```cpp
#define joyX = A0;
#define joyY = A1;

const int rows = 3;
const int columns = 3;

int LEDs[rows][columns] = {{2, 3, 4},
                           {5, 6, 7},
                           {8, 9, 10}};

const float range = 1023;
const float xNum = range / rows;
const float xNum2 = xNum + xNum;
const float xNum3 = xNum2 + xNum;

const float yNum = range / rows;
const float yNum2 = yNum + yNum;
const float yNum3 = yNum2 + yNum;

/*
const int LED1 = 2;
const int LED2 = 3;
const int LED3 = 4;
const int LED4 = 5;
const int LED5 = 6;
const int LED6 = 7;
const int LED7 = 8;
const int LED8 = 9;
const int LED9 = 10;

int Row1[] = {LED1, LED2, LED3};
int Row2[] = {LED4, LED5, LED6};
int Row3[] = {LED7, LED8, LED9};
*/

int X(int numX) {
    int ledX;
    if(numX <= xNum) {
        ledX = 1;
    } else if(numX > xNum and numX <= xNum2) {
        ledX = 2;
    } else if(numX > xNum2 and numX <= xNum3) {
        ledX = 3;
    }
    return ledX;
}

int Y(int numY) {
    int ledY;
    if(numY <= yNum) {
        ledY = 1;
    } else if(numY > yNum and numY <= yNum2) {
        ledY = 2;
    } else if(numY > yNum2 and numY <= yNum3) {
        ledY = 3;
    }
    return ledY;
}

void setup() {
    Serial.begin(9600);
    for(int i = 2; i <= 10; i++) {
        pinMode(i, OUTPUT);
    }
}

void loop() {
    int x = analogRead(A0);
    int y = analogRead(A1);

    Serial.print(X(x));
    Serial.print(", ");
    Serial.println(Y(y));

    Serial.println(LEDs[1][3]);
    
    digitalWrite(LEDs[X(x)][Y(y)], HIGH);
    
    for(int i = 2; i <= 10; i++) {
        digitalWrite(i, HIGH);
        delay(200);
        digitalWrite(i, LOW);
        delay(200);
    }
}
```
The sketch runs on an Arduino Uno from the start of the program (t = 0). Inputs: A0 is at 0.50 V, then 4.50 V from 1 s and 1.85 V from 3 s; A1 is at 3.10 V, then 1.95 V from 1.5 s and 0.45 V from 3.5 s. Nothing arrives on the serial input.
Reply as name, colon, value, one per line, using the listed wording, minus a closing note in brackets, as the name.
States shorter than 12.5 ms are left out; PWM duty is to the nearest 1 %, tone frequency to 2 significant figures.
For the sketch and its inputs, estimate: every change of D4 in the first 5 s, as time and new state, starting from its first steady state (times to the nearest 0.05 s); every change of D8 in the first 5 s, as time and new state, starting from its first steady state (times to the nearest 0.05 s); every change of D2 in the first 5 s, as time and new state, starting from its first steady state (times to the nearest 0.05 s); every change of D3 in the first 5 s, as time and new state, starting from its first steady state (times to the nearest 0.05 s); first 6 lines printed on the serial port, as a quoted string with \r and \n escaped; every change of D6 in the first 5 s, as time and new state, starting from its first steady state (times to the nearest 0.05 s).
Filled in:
every change of D4 in the first 5 s, as time and new state, starting from its first steady state: 0 s low; 0.8 s high; 1 s low; 4.4 s high; 4.6 s low
every change of D8 in the first 5 s, as time and new state, starting from its first steady state: 0 s low; 2.4 s high; 2.6 s low
every change of D2 in the first 5 s, as time and new state, starting from its first steady state: 0 s high; 0.2 s low; 3.6 s high; 3.8 s low
every change of D3 in the first 5 s, as time and new state, starting from its first steady state: 0 s low; 0.4 s high; 0.6 s low; 4 s high; 4.2 s low
first 6 lines printed on the serial port, as a quoted string with \r and \n escaped: "1, 2\r\n8\r\n2, 1\r\n8\r\n2, 1\r\n8\r\n"
every change of D6 in the first 5 s, as time and new state, starting from its first steady state: 0 s low; 1.6 s high; 1.8 s low
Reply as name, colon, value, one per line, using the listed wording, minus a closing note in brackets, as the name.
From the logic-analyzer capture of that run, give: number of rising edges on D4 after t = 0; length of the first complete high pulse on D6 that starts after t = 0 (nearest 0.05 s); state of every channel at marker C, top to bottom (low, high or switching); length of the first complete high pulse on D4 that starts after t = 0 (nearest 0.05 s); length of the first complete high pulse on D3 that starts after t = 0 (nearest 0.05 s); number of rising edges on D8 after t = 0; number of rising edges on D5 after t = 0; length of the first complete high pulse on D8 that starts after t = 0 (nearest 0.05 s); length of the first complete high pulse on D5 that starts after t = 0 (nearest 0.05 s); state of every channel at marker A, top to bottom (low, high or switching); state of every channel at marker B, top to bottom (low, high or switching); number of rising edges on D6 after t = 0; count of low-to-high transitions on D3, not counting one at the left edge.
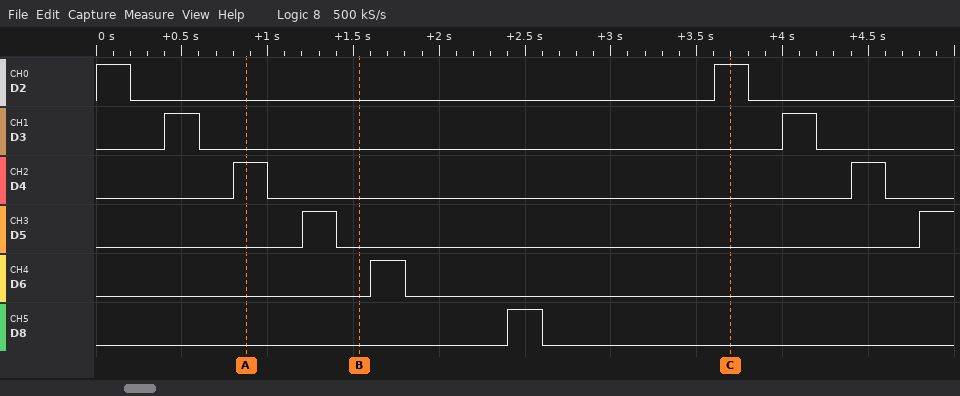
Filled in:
number of rising edges on D4 after t = 0: 2
length of the first complete high pulse on D6 that starts after t = 0: 0.20 s
state of every channel at marker C, top to bottom: D2 high, D3 low, D4 low, D5 low, D6 low, D8 low
length of the first complete high pulse on D4 that starts after t = 0: 0.20 s
length of the first complete high pulse on D3 that starts after t = 0: 0.20 s
number of rising edges on D8 after t = 0: 1
number of rising edges on D5 after t = 0: 2
length of the first complete high pulse on D8 that starts after t = 0: 0.20 s
length of the first complete high pulse on D5 that starts after t = 0: 0.20 s
state of every channel at marker A, top to bottom: D2 low, D3 low, D4 high, D5 low, D6 low, D8 low
state of every channel at marker B, top to bottom: D2 low, D3 low, D4 low, D5 low, D6 low, D8 low
number of rising edges on D6 after t = 0: 1
count of low-to-high transitions on D3, not counting one at the left edge: 2
